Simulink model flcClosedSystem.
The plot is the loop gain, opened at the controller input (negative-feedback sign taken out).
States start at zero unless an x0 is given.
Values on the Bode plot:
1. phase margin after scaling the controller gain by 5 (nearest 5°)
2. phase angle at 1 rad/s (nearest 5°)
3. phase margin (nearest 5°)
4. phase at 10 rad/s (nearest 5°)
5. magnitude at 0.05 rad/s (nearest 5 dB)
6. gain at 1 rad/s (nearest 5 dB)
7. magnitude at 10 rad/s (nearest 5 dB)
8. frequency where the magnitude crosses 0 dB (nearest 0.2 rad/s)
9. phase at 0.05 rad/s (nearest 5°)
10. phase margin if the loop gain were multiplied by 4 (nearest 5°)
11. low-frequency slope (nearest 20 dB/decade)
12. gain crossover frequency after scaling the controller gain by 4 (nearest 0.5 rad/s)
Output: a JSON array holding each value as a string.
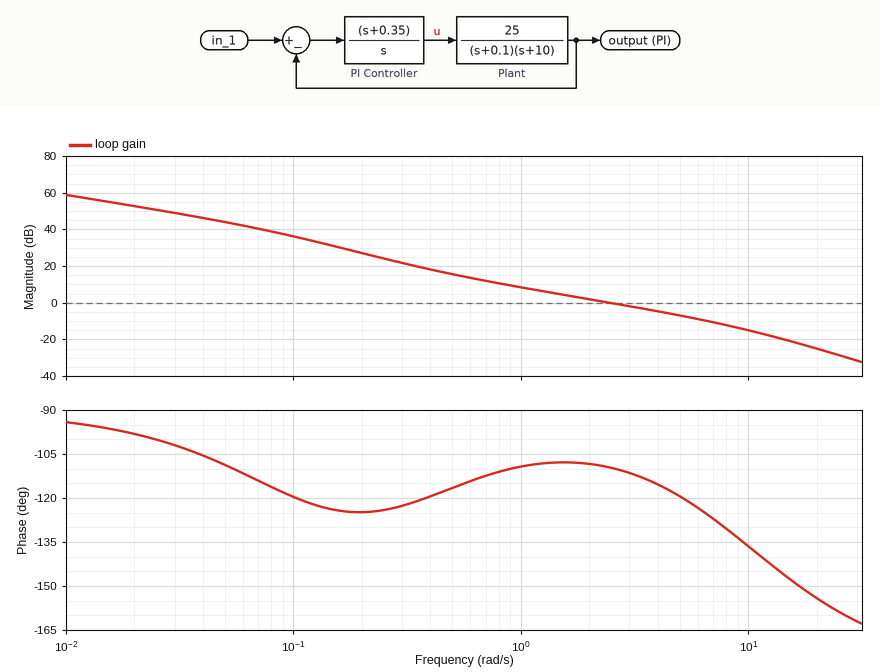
["45°", "-110°", "70°", "-135°", "45 dB", "10 dB", "-15 dB", "2.4 rad/s", "-110°", "50°", "-20 dB/decade", "8.0 rad/s"]
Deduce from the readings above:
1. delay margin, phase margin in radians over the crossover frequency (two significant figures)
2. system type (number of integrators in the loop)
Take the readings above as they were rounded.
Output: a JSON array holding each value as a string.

["0.51 s", "1"]
